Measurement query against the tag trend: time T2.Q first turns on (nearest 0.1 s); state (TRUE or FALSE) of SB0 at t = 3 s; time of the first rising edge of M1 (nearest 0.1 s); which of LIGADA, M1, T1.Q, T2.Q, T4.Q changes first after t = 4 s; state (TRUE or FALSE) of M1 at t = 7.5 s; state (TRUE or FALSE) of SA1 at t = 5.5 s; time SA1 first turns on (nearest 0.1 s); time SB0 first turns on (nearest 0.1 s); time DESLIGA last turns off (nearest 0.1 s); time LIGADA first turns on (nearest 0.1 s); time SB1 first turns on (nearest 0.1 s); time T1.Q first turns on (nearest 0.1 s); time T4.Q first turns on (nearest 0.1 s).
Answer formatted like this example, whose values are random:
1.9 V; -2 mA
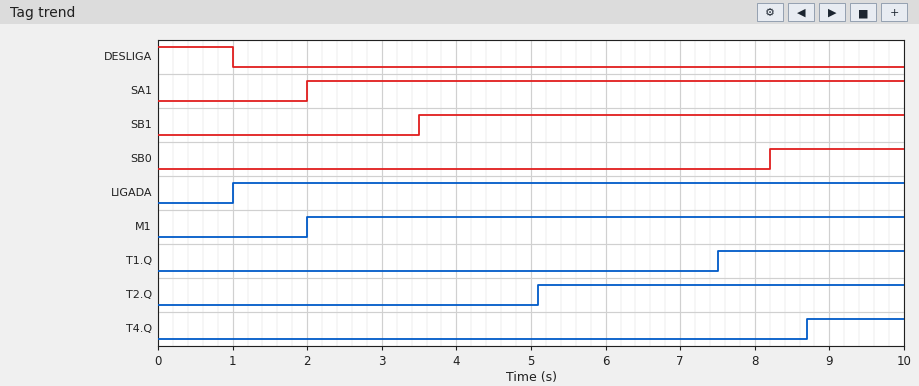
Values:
5.1 s; FALSE; 2.0 s; T2.Q; TRUE; TRUE; 2.0 s; 8.2 s; 1.0 s; 1.0 s; 3.5 s; 7.5 s; 8.7 s
